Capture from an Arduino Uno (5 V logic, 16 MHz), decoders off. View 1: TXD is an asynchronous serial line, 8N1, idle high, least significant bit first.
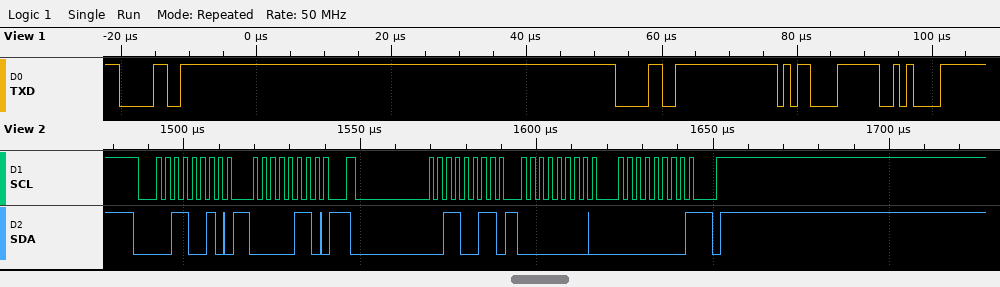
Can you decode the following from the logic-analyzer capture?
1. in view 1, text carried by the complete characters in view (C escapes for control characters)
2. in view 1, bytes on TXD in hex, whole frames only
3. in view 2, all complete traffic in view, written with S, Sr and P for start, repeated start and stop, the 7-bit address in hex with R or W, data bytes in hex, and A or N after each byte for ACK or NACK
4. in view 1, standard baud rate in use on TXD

"00\r\n"
30 30 0D 0A
S 19W A 06 A Sr 19R A 00 A 00 N P
1000000 baud
